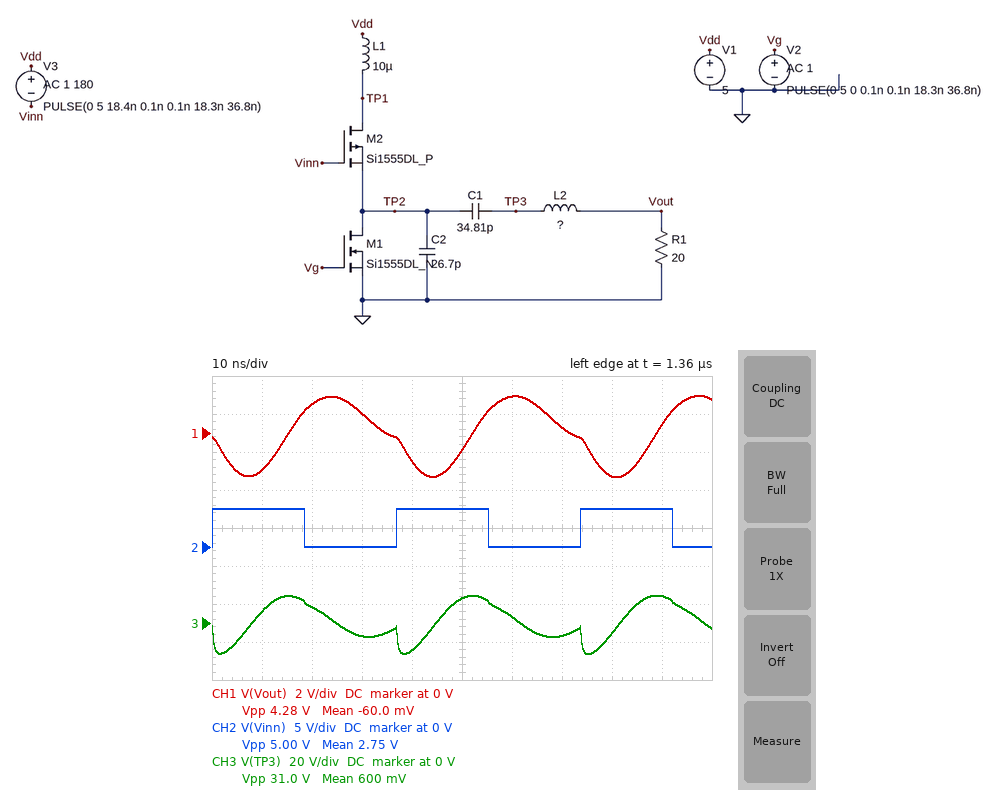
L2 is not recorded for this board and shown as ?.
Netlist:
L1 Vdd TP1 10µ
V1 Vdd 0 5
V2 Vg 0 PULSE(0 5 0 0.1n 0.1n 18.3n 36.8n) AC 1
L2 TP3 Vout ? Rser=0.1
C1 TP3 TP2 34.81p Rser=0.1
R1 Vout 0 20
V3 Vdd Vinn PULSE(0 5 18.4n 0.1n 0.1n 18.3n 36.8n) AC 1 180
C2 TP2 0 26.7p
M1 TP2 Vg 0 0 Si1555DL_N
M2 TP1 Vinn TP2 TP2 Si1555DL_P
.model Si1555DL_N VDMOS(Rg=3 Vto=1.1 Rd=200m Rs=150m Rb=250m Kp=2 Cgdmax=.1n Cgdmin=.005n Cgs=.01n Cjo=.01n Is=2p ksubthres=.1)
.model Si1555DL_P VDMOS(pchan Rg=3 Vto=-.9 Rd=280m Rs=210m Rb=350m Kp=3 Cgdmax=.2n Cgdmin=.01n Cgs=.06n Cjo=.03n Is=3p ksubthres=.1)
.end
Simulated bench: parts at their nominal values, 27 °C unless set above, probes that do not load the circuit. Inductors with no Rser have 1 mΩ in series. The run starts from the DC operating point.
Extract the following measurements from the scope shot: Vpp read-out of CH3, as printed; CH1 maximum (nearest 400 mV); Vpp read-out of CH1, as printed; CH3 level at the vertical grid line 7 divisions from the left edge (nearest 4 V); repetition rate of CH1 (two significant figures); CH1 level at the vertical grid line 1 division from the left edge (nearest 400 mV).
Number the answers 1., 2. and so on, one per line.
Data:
1. 31.0 V
2. 2.0 V
3. 4.28 V
4. -8 V
5. 27 MHz
6. -2.0 V
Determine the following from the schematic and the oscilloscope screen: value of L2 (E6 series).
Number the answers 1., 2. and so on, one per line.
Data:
1. 680 nH
